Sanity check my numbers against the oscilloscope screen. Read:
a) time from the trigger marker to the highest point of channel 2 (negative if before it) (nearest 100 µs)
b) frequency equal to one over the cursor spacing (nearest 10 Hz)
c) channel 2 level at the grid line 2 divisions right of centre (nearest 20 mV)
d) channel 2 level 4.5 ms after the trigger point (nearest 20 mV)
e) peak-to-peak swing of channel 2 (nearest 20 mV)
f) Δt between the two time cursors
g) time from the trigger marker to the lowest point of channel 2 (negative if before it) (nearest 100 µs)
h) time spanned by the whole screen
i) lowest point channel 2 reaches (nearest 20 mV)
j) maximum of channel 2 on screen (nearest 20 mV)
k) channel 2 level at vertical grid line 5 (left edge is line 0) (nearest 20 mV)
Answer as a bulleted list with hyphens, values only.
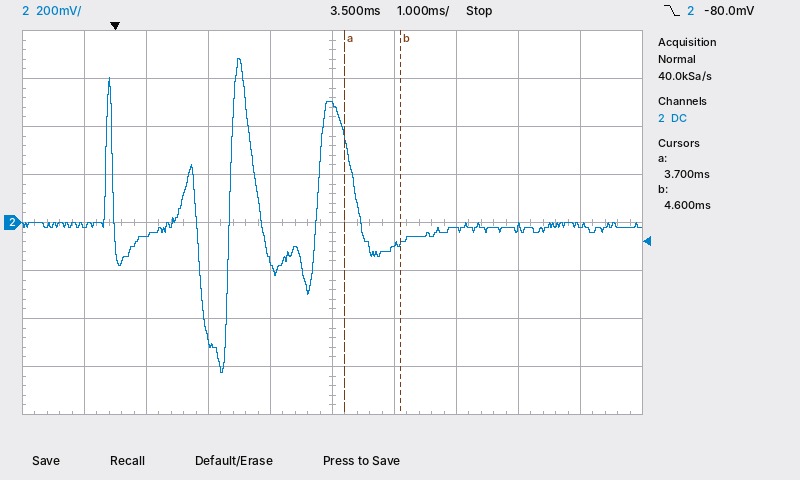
- +2.0 ms
- 1.11 kHz
- -20 mV
- -100 mV
- 1.30 V
- 900 µs
- +1.7 ms
- 10 ms
- -620 mV
- 680 mV
- 500 mV
